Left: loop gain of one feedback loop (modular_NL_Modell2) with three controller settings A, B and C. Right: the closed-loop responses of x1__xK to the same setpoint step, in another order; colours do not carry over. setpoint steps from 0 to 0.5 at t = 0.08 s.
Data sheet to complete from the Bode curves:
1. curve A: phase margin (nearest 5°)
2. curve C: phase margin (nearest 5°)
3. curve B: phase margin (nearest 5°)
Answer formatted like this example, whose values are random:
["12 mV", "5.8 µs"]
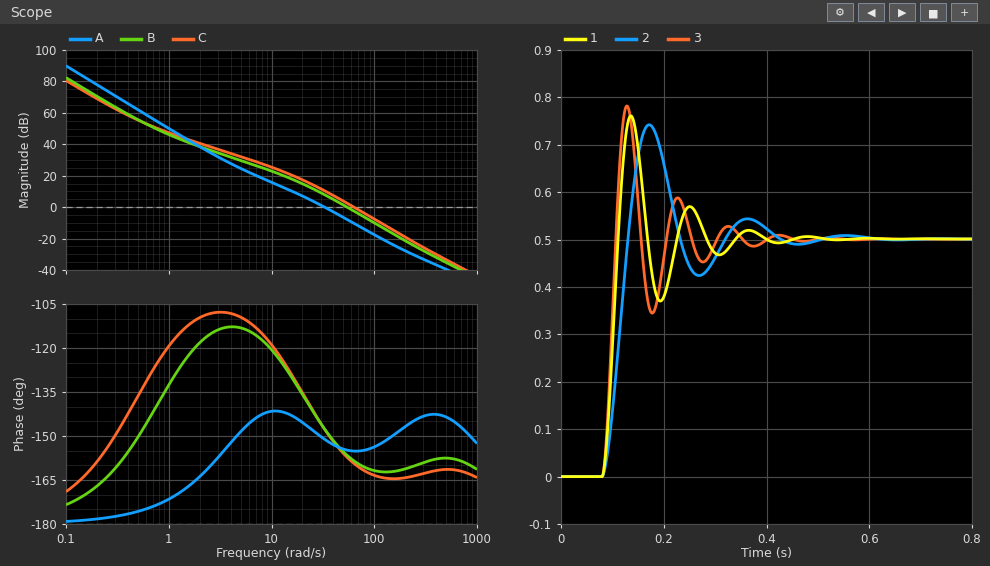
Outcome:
["30°", "20°", "25°"]
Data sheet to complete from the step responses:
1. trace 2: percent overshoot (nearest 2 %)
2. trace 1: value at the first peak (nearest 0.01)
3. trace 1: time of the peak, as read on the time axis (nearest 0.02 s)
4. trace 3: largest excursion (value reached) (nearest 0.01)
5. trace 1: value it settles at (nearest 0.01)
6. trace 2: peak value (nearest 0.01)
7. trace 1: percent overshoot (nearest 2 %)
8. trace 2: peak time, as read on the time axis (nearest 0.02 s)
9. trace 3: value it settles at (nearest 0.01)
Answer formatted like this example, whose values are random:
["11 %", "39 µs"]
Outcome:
["48 %", "0.76", "0.14 s", "0.78", "0.50", "0.74", "52 %", "0.18 s", "0.50"]
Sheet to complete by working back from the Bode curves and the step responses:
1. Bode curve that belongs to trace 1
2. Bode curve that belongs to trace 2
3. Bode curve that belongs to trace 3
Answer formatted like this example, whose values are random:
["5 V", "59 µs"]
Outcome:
["B", "A", "C"]
